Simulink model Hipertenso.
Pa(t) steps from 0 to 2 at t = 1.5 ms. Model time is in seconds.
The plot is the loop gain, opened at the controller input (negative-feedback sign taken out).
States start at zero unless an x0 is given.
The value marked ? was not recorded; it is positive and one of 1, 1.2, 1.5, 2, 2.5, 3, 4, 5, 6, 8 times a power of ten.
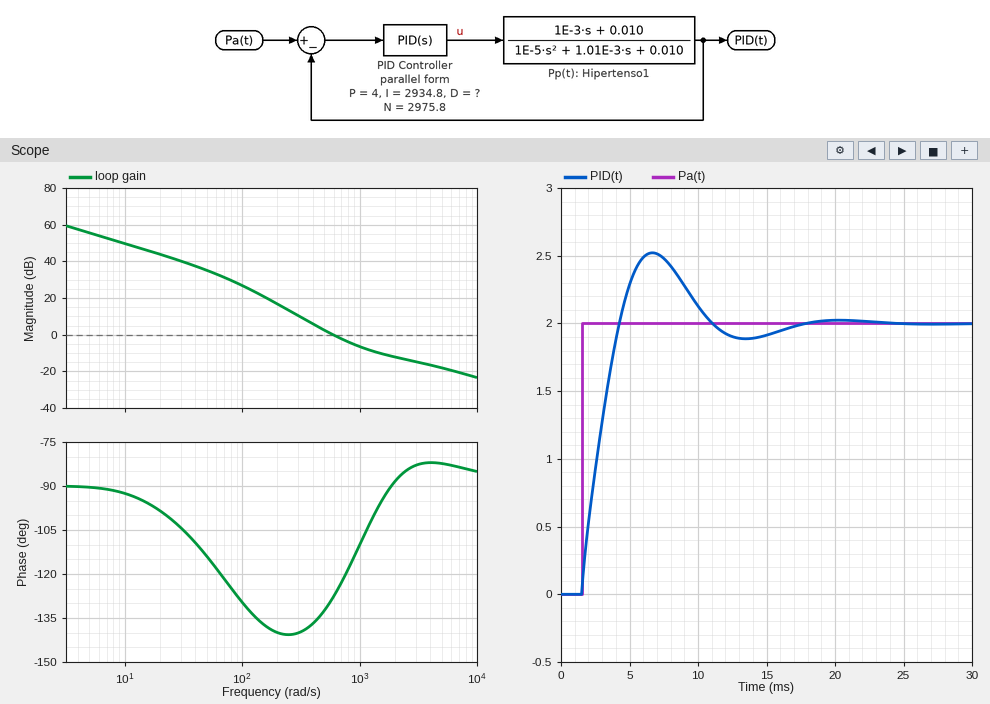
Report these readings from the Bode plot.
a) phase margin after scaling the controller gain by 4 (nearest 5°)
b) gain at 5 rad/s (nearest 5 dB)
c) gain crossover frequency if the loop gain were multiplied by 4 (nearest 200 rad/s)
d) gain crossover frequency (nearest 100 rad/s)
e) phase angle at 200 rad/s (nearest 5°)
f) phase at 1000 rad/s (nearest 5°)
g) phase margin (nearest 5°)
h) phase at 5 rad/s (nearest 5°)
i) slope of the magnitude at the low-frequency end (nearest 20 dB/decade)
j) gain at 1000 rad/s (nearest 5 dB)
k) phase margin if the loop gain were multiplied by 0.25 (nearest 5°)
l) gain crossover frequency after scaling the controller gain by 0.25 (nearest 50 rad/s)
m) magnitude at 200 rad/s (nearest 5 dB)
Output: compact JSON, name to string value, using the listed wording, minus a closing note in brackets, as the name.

{"phase margin after scaling the controller gain by 4": "90°", "gain at 5 rad/s": "55 dB", "gain crossover frequency if the loop gain were multiplied by 4": "2000 rad/s", "gain crossover frequency": "600 rad/s", "phase angle at 200 rad/s": "-140°", "phase at 1000 rad/s": "-110°", "phase margin": "50°", "phase at 5 rad/s": "-90°", "slope of the magnitude at the low-frequency end": "-20 dB/decade", "gain at 1000 rad/s": "-5 dB", "phase margin if the loop gain were multiplied by 0.25": "40°", "gain crossover frequency after scaling the controller gain by 0.25": "250 rad/s", "magnitude at 200 rad/s": "15 dB"}
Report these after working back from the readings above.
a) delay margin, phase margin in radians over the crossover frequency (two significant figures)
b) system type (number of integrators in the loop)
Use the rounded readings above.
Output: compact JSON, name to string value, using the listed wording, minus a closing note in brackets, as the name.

{"delay margin, phase margin in radians over the crossover frequency": "0.0015 s", "system type": "1"}
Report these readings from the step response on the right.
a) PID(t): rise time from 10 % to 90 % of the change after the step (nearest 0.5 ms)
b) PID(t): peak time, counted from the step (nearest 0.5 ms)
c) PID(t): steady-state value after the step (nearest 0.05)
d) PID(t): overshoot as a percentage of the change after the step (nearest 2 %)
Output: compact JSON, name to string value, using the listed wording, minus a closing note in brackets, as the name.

{"PID(t): rise time from 10 % to 90 % of the change after the step": "2.0 ms", "PID(t): peak time, counted from the step": "5.0 ms", "PID(t): steady-state value after the step": "2.00", "PID(t): overshoot as a percentage of the change after the step": "26 %"}
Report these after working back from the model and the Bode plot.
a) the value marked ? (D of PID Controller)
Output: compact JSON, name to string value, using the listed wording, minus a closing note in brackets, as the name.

{"the value marked ?": "0.001"}
